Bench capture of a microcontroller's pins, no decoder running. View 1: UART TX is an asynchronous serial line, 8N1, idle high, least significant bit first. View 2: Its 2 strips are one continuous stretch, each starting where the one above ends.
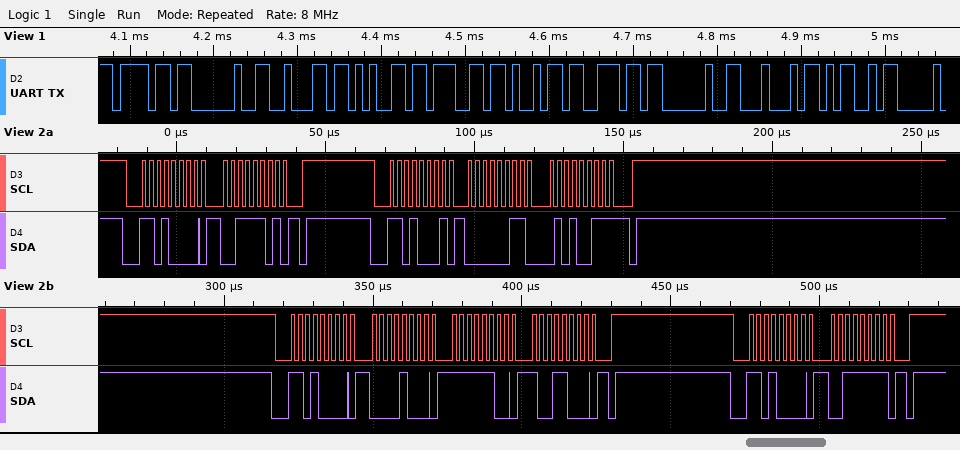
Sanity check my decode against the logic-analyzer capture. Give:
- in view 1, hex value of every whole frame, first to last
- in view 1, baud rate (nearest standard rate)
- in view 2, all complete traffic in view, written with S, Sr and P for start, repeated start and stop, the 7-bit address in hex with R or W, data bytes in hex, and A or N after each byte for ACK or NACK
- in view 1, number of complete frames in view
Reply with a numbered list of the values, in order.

1. 6F 20 62 65 67 69 6E 20 44 4D
2. 115200 baud
3. S 68W A 3D A P S 68R A 03 A 53 N P S 68W A 08 A FC A 98 A P S 68W A 3F A P
4. 10
